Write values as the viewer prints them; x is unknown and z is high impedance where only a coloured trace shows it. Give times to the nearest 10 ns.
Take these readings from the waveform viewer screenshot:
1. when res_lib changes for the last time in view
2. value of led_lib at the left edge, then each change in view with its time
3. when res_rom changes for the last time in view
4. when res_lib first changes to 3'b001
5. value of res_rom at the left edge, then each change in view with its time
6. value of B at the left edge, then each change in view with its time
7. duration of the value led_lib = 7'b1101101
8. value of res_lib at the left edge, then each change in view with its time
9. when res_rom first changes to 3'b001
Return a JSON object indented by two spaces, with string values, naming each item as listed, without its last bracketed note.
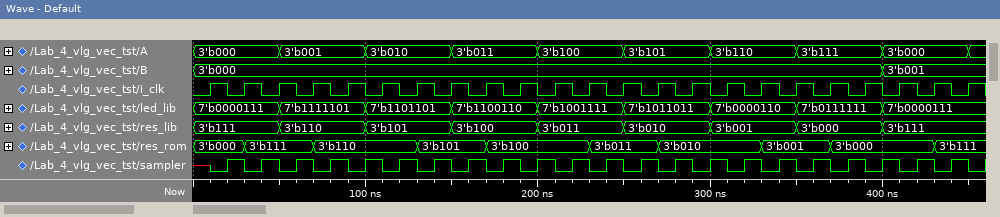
{
  "when res_lib changes for the last time in view": "400 ns",
  "value of led_lib at the left edge, then each change in view with its time": "7'b0000111, 7'b1111101 at 50 ns, 7'b1101101 at 100 ns, 7'b1100110 at 150 ns, 7'b1001111 at 200 ns, 7'b1011011 at 250 ns, 7'b0000110 at 300 ns, 7'b0111111 at 350 ns, 7'b0000111 at 400 ns",
  "when res_rom changes for the last time in view": "430 ns",
  "when res_lib first changes to 3'b001": "300 ns",
  "value of res_rom at the left edge, then each change in view with its time": "3'b000, 3'b111 at 30 ns, 3'b110 at 70 ns, 3'b101 at 130 ns, 3'b100 at 170 ns, 3'b011 at 230 ns, 3'b010 at 270 ns, 3'b001 at 330 ns, 3'b000 at 370 ns, 3'b111 at 430 ns",
  "value of B at the left edge, then each change in view with its time": "3'b000, 3'b001 at 400 ns",
  "duration of the value led_lib = 7'b1101101": "50 ns",
  "value of res_lib at the left edge, then each change in view with its time": "3'b111, 3'b110 at 50 ns, 3'b101 at 100 ns, 3'b100 at 150 ns, 3'b011 at 200 ns, 3'b010 at 250 ns, 3'b001 at 300 ns, 3'b000 at 350 ns, 3'b111 at 400 ns",
  "when res_rom first changes to 3'b001": "330 ns"
}
